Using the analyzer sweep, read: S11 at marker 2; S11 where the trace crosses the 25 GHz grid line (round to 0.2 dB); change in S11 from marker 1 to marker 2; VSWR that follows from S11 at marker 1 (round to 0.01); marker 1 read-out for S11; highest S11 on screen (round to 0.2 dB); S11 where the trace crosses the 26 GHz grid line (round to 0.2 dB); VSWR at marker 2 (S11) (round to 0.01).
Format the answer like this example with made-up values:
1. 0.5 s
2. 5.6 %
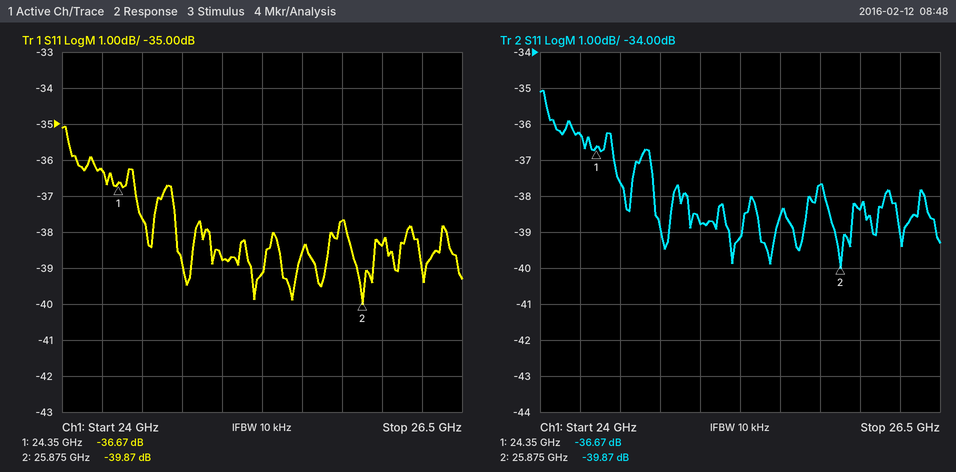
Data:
1. -39.87 dB
2. -38.8 dB
3. -3.20 dB
4. 1.03
5. -36.67 dB
6. -35.0 dB
7. -38.4 dB
8. 1.02
